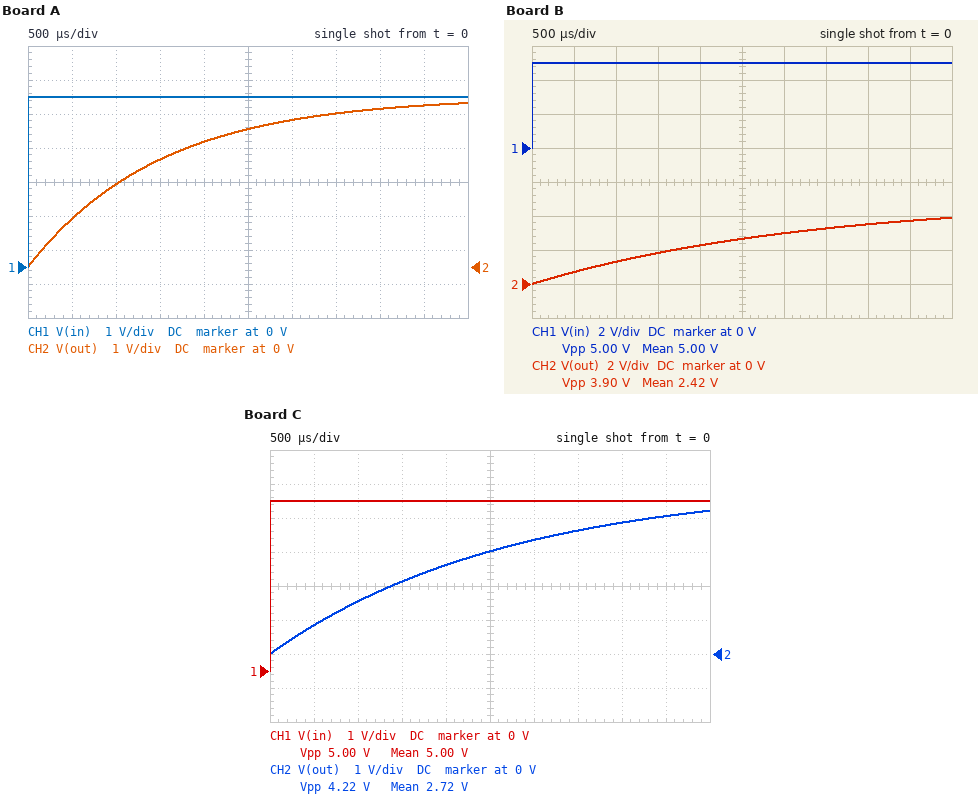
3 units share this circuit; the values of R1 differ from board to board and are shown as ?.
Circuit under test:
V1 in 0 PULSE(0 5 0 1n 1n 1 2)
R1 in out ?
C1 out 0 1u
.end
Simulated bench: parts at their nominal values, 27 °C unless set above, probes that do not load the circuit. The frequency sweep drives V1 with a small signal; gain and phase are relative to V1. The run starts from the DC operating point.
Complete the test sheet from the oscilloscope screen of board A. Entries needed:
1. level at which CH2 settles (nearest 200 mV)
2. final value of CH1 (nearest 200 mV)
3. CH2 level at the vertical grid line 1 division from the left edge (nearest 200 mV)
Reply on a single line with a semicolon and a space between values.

4.8 V; 5.0 V; 1.4 V
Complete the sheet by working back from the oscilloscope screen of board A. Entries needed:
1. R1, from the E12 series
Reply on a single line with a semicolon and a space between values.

1.5 kΩ
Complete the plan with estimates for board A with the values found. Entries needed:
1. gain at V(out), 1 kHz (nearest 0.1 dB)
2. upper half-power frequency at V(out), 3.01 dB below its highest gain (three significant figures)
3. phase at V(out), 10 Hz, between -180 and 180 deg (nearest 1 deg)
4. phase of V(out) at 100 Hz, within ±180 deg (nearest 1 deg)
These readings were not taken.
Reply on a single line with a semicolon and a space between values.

-19.5 dB; 106 Hz; -5 deg; -43 deg
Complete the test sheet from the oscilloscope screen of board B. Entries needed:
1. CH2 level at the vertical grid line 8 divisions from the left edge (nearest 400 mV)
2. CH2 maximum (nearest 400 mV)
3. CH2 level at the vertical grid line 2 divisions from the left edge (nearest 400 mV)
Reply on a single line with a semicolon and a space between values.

3.6 V; 4.0 V; 1.2 V
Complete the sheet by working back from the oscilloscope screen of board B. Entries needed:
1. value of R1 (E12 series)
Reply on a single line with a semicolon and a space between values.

3.3 kΩ
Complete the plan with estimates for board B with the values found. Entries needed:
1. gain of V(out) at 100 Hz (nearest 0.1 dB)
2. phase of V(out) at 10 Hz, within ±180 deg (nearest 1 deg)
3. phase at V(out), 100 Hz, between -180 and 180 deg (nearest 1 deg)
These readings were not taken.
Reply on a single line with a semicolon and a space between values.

-7.2 dB; -12 deg; -64 deg
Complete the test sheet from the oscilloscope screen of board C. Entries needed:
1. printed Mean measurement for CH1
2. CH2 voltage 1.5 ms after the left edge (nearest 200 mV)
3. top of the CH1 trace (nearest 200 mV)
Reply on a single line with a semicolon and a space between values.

5.00 V; 2.2 V; 5.0 V
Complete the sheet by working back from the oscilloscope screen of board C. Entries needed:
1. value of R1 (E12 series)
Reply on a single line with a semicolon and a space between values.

2.7 kΩ
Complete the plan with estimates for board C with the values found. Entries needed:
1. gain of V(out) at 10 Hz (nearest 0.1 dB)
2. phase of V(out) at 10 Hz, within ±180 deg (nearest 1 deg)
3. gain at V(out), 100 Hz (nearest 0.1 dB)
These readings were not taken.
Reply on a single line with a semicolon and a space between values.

-0.1 dB; -10 deg; -5.9 dB
